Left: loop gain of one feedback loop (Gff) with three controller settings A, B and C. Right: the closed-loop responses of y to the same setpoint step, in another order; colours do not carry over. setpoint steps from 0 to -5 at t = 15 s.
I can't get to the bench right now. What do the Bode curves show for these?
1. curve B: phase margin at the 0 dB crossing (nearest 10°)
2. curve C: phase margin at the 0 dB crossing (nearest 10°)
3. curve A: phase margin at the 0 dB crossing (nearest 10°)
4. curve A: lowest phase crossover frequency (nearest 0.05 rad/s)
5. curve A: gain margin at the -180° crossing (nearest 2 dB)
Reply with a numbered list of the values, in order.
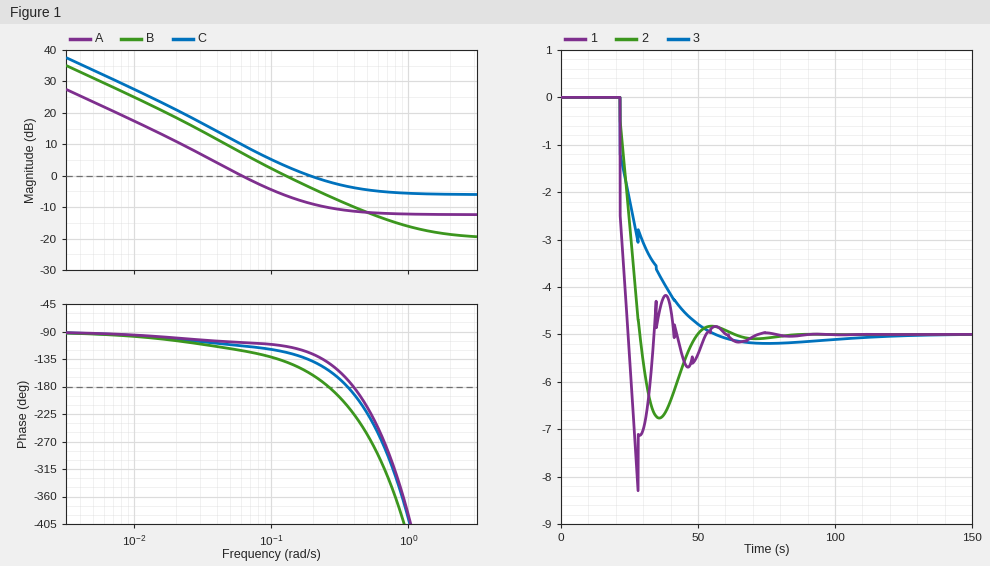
1. 40°
2. 40°
3. 70°
4. 0.40 rad/s
5. 12 dB
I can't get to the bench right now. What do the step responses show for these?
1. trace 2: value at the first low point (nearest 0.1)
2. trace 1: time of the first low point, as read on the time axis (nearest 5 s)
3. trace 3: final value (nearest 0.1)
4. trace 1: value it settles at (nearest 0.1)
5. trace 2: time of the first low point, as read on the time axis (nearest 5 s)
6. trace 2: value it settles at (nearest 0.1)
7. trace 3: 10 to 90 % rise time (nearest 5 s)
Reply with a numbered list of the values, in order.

1. -6.8
2. 30 s
3. -5.0
4. -5.0
5. 35 s
6. -5.0
7. 25 s
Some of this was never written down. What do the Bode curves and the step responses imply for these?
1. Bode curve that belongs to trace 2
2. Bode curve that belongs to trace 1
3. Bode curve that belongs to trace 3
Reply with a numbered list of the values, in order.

1. B
2. C
3. A
